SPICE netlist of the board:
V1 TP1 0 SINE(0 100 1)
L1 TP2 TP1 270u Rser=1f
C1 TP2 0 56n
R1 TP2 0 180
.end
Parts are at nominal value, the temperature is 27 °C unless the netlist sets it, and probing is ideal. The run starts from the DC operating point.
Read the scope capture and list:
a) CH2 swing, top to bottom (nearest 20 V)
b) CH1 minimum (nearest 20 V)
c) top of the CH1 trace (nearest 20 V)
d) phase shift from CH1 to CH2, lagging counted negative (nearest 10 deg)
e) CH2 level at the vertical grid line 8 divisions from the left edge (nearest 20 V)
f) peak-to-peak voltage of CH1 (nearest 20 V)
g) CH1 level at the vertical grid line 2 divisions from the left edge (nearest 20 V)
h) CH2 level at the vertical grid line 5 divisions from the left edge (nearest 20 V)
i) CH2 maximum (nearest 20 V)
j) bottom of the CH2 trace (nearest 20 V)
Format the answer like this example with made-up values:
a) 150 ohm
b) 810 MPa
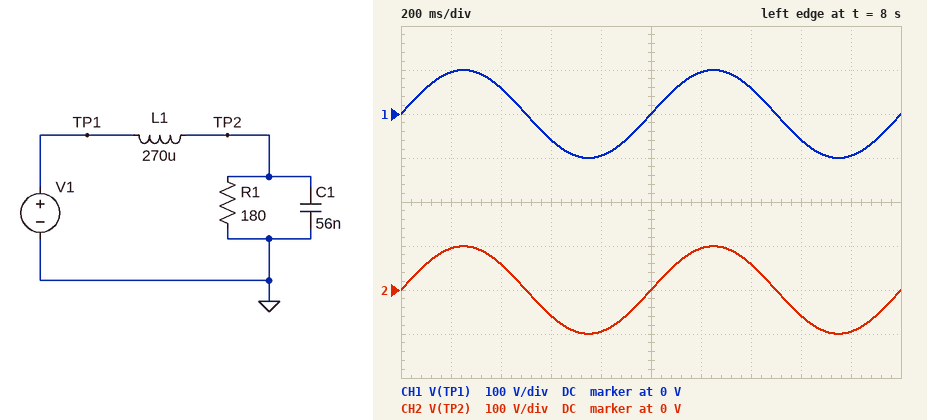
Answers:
a) 200 V
b) -100 V
c) 100 V
d) 0 deg
e) -60 V
f) 200 V
g) 60 V
h) 0 V
i) 100 V
j) -100 V
